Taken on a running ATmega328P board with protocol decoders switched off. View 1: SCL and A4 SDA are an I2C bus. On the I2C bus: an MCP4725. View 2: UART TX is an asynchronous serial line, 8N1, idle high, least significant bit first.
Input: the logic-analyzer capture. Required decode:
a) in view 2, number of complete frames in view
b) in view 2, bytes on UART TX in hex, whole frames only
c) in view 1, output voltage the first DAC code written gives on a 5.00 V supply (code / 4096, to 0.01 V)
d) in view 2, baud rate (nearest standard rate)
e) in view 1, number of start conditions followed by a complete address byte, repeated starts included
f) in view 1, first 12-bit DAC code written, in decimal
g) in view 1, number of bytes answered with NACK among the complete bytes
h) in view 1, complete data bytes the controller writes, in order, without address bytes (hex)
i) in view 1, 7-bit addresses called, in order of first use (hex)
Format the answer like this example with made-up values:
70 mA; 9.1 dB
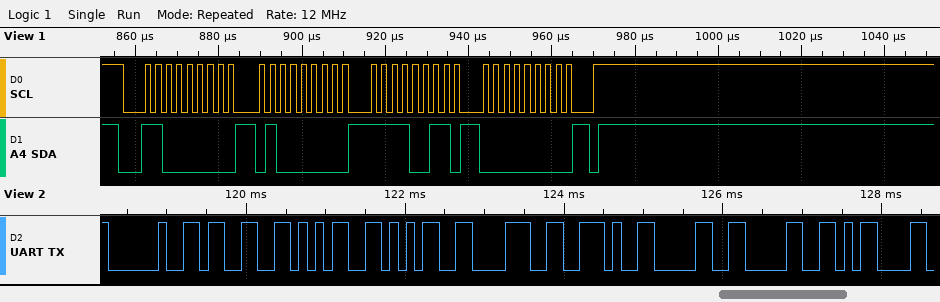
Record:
9; 20 33 35 35 38 2E 30 30 0D; 4.75 V; 9600 baud; 1; 3888; 0; 40 F3 00; 0x60
